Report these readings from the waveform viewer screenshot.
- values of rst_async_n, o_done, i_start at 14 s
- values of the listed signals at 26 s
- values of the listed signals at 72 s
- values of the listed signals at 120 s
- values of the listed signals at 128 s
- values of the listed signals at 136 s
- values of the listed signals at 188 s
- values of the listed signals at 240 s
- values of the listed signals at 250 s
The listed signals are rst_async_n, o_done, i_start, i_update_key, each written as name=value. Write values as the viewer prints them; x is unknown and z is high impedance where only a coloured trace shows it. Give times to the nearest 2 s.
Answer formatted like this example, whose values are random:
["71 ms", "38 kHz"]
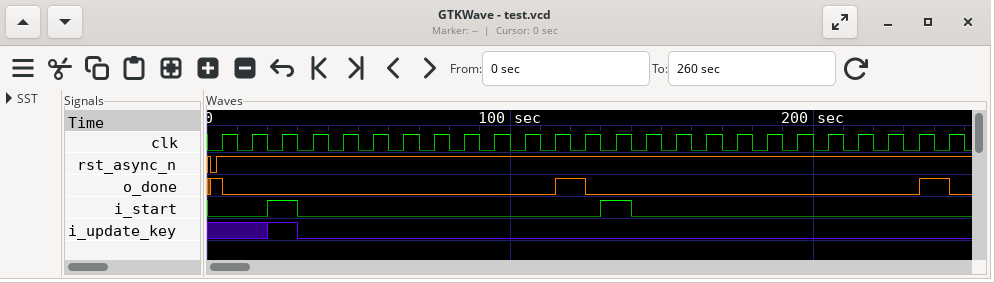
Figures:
["rst_async_n=1, o_done=0, i_start=0", "rst_async_n=1, o_done=0, i_start=1, i_update_key=1", "rst_async_n=1, o_done=0, i_start=0, i_update_key=0", "rst_async_n=1, o_done=1, i_start=0, i_update_key=0", "rst_async_n=1, o_done=0, i_start=0, i_update_key=0", "rst_async_n=1, o_done=0, i_start=1, i_update_key=0", "rst_async_n=1, o_done=0, i_start=0, i_update_key=0", "rst_async_n=1, o_done=1, i_start=0, i_update_key=0", "rst_async_n=1, o_done=0, i_start=0, i_update_key=0"]
